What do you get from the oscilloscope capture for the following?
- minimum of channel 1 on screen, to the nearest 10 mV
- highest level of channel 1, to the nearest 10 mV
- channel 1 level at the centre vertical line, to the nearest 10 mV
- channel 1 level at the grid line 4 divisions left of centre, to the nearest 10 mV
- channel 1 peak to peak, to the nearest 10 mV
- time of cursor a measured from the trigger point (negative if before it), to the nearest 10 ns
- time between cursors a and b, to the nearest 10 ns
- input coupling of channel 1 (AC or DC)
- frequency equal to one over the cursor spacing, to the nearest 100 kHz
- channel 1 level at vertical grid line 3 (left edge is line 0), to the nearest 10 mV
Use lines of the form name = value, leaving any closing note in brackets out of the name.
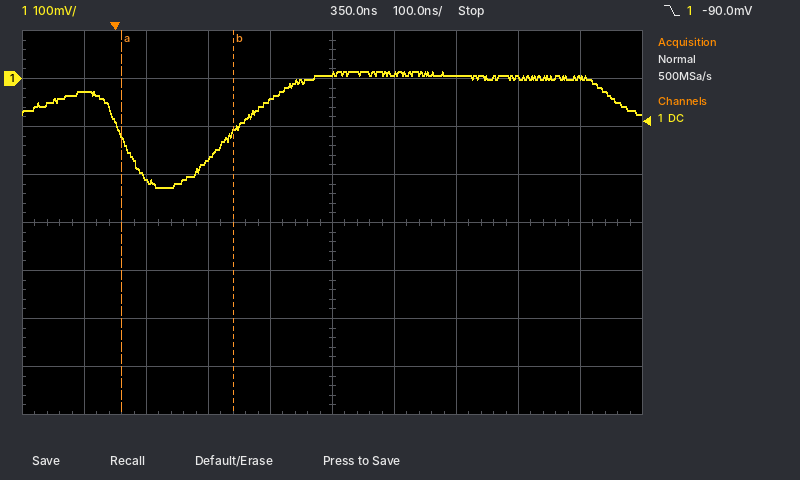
minimum of channel 1 on screen, to the nearest 10 mV = -230 mV
highest level of channel 1, to the nearest 10 mV = 10 mV
channel 1 level at the centre vertical line, to the nearest 10 mV = 10 mV
channel 1 level at the grid line 4 divisions left of centre, to the nearest 10 mV = -30 mV
channel 1 peak to peak, to the nearest 10 mV = 240 mV
time of cursor a measured from the trigger point (negative if before it), to the nearest 10 ns = +10 ns
time between cursors a and b, to the nearest 10 ns = 180 ns
input coupling of channel 1 = DC
frequency equal to one over the cursor spacing, to the nearest 100 kHz = 5.6 MHz
channel 1 level at vertical grid line 3 (left edge is line 0), to the nearest 10 mV = -170 mV
